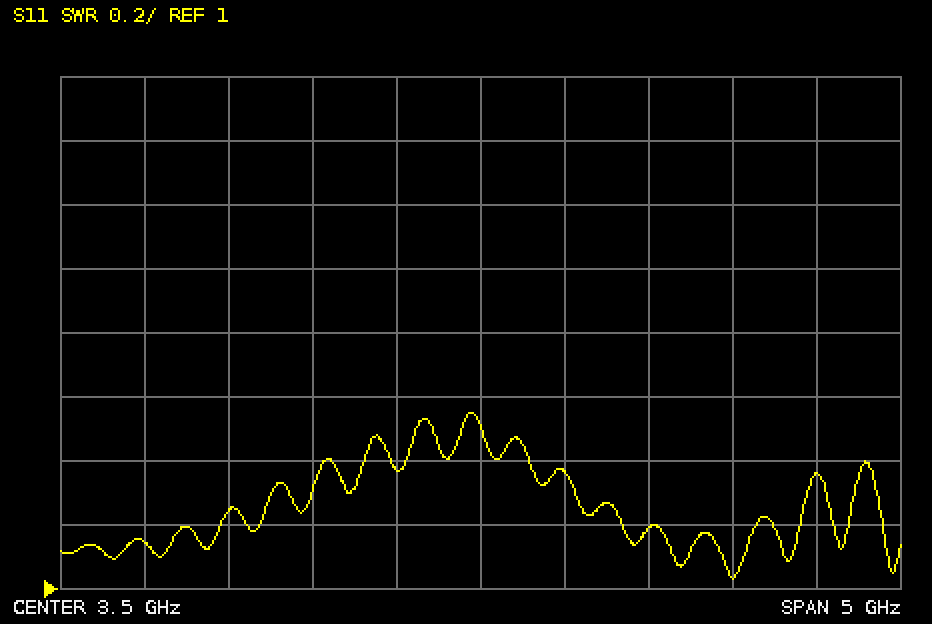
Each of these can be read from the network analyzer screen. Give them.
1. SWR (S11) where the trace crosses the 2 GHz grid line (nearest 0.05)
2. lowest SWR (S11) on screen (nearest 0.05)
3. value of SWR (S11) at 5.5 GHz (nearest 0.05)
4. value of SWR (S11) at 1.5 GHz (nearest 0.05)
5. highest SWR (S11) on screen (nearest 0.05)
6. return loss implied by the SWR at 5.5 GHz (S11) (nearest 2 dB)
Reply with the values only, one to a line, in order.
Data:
1.25
1.05
1.35
1.15
1.55
16 dB
